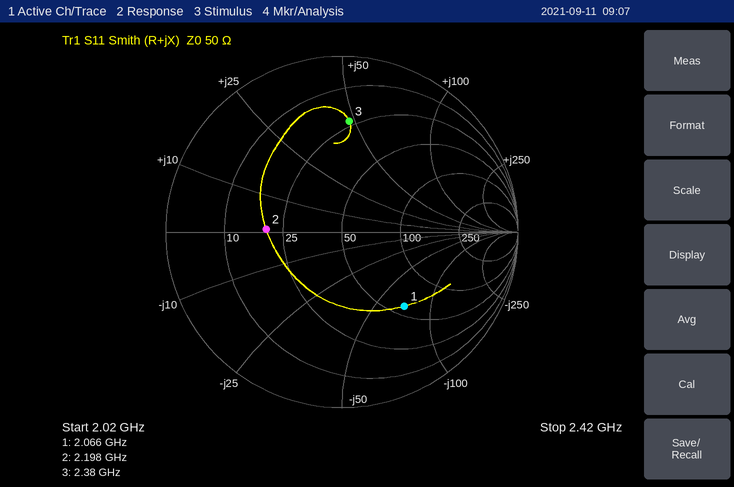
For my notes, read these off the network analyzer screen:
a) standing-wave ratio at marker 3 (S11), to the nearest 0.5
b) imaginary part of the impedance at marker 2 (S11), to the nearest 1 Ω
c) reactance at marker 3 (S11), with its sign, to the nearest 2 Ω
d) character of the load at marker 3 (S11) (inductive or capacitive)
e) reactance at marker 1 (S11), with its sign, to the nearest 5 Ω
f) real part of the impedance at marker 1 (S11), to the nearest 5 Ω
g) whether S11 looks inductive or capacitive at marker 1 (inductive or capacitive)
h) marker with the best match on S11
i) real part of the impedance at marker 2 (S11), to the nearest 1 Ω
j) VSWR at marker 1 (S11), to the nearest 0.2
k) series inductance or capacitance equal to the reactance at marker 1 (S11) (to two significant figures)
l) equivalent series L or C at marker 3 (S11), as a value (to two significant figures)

4.5
+1 Ω
+48 Ω
inductive
-70 Ω
60 Ω
capacitive
marker 2
20 Ω
3.4
1.1 pF
3.2 nH
